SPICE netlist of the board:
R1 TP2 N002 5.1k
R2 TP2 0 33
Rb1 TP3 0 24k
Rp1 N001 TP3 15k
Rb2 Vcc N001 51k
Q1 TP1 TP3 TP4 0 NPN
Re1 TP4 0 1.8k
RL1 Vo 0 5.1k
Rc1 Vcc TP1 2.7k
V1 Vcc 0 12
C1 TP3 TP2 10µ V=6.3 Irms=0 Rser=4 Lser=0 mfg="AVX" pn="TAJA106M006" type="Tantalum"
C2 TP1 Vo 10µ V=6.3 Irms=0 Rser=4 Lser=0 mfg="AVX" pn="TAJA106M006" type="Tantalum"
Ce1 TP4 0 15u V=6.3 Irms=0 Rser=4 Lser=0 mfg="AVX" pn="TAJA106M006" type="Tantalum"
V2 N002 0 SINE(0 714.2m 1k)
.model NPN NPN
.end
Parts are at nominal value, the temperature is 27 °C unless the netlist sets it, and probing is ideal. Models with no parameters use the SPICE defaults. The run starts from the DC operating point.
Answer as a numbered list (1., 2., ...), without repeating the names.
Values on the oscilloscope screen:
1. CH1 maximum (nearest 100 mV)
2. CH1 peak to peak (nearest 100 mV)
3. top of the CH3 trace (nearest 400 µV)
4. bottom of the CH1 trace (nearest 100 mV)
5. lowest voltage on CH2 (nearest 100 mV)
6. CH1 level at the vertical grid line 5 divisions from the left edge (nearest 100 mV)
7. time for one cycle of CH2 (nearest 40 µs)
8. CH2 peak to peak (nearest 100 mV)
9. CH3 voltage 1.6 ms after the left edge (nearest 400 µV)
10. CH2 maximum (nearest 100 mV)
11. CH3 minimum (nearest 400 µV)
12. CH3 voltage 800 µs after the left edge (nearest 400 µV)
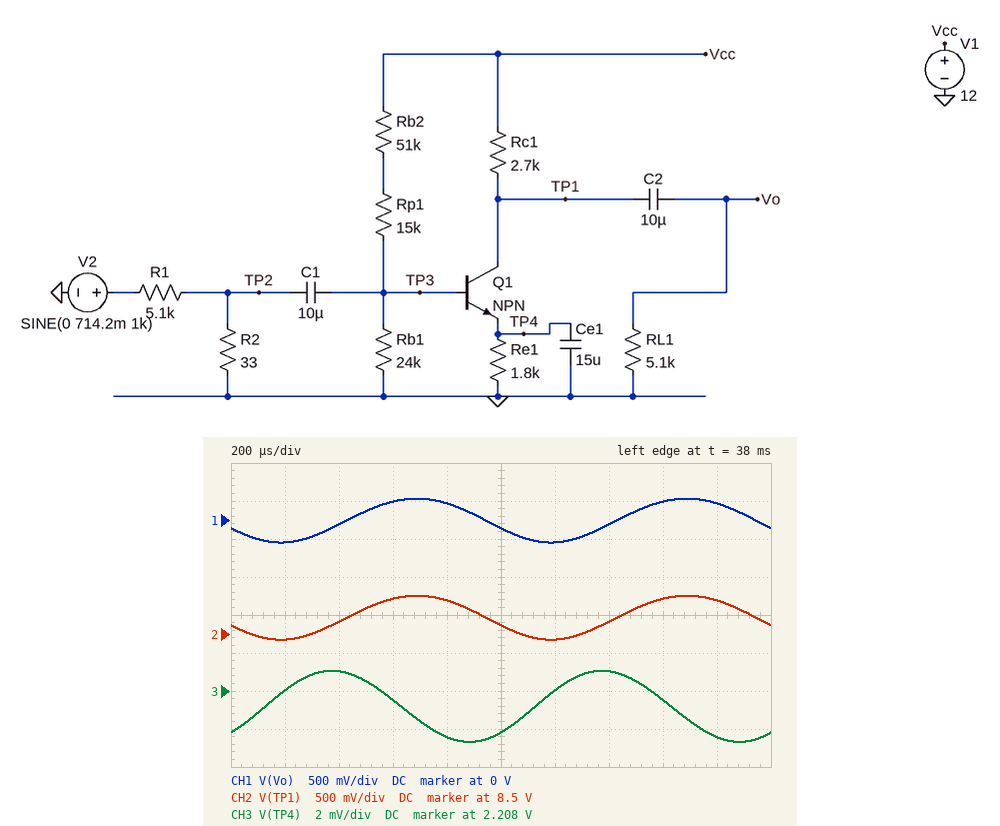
1. 300 mV
2. 600 mV
3. 2.2092 V
4. -300 mV
5. 8.4 V
6. -100 mV
7. 1.00 ms
8. 600 mV
9. 2.2076 V
10. 9.0 V
11. 2.2052 V
12. 2.2056 V
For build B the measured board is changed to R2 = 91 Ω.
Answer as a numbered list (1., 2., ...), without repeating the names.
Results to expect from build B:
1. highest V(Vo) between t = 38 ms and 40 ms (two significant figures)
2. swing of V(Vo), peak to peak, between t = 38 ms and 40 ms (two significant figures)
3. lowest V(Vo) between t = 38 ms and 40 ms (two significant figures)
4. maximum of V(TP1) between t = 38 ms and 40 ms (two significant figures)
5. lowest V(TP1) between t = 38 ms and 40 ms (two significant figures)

1. 710 mV
2. 1.5 V
3. -820 mV
4. 9.4 V
5. 7.9 V
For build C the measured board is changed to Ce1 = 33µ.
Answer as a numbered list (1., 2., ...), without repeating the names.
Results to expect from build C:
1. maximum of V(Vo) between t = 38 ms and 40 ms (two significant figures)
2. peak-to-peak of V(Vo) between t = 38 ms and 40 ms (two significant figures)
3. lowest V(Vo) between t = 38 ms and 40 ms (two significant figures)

1. 300 mV
2. 620 mV
3. -320 mV
